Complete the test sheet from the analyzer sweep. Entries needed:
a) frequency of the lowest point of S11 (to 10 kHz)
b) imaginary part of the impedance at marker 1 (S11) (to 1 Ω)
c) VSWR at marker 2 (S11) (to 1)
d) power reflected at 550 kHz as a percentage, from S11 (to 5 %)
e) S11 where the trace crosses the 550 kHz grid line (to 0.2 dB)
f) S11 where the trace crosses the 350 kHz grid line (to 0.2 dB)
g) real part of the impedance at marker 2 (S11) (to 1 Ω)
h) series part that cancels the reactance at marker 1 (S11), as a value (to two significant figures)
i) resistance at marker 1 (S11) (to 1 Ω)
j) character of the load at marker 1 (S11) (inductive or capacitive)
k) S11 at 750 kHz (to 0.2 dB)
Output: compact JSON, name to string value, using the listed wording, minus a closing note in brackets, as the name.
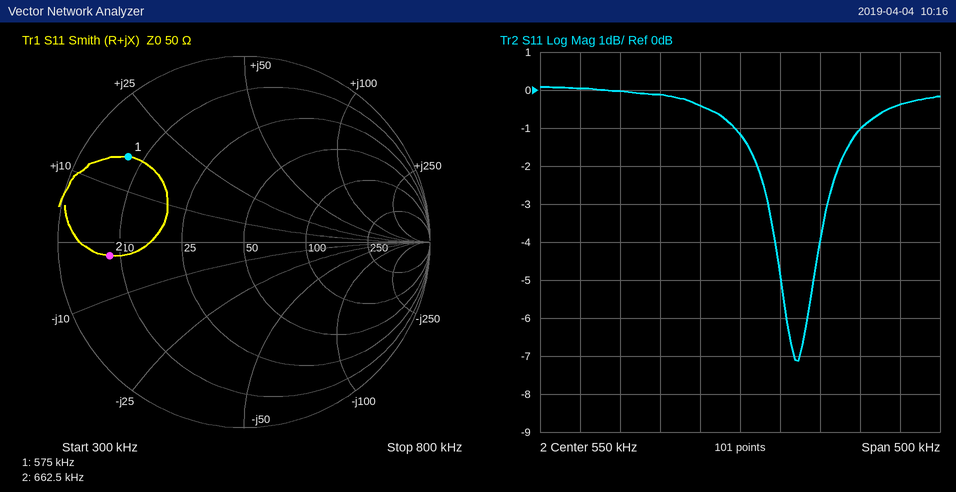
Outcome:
{"frequency of the lowest point of S11": "620 kHz", "imaginary part of the impedance at marker 1 (S11)": "+16 Ω", "VSWR at marker 2 (S11)": "6", "power reflected at 550 kHz as a percentage, from S11": "75 %", "S11 where the trace crosses the 550 kHz grid line": "-1.2 dB", "S11 where the trace crosses the 350 kHz grid line": "0.0 dB", "real part of the impedance at marker 2 (S11)": "8 Ω", "series part that cancels the reactance at marker 1 (S11), as a value": "17 nF", "resistance at marker 1 (S11)": "7 Ω", "character of the load at marker 1 (S11)": "inductive", "S11 at 750 kHz": "-0.4 dB"}
